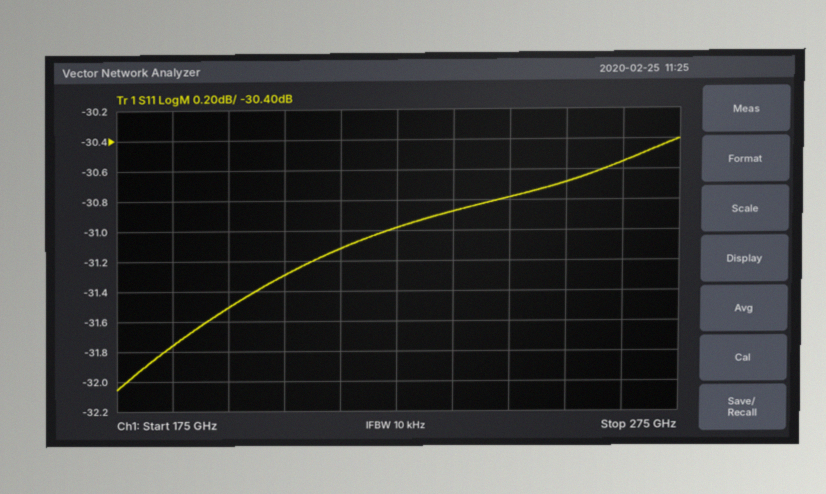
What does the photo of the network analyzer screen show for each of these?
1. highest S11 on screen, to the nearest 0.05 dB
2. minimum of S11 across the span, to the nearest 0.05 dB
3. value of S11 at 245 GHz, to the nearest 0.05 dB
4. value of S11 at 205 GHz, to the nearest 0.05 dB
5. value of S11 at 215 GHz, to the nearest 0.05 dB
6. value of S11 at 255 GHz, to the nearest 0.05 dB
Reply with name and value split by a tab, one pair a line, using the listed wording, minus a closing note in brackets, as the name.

highest S11 on screen, to the nearest 0.05 dB	-30.40 dB
minimum of S11 across the span, to the nearest 0.05 dB	-32.05 dB
value of S11 at 245 GHz, to the nearest 0.05 dB	-30.80 dB
value of S11 at 205 GHz, to the nearest 0.05 dB	-31.30 dB
value of S11 at 215 GHz, to the nearest 0.05 dB	-31.10 dB
value of S11 at 255 GHz, to the nearest 0.05 dB	-30.70 dB
